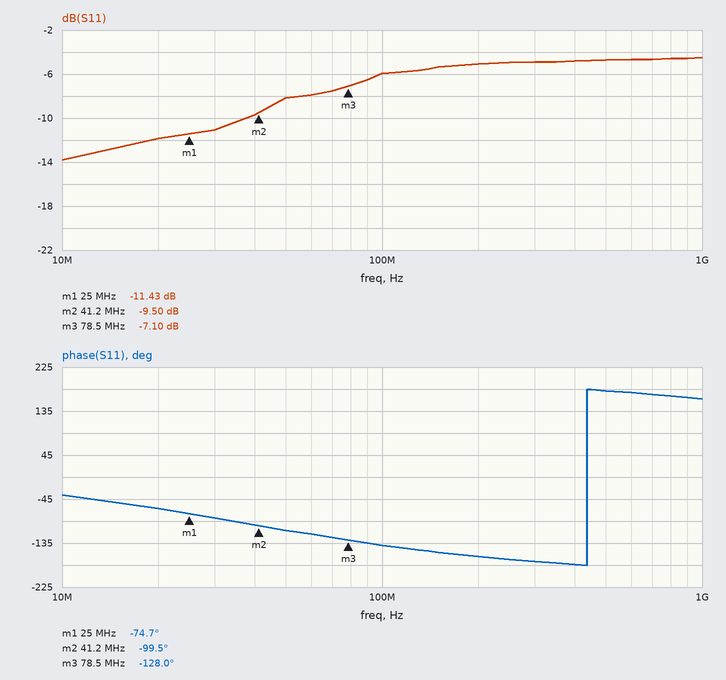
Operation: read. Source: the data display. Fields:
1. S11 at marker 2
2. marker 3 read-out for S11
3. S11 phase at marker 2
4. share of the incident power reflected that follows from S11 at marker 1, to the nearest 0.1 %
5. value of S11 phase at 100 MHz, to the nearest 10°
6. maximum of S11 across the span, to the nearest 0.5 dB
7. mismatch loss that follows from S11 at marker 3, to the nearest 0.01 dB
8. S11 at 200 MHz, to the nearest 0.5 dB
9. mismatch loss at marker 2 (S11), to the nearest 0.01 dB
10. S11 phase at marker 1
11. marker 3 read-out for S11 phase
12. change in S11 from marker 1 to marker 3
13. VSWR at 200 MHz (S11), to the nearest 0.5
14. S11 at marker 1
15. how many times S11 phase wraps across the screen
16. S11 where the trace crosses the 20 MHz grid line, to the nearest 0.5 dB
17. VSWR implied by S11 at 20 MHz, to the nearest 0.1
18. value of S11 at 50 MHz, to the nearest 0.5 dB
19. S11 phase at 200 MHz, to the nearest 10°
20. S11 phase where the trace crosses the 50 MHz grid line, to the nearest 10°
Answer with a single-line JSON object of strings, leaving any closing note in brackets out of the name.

{"S11 at marker 2": "-9.50 dB", "marker 3 read-out for S11": "-7.10 dB", "S11 phase at marker 2": "-99.5°", "share of the incident power reflected that follows from S11 at marker 1, to the nearest 0.1 %": "7.2 %", "value of S11 phase at 100 MHz, to the nearest 10°": "-140°", "maximum of S11 across the span, to the nearest 0.5 dB": "-4.5 dB", "mismatch loss that follows from S11 at marker 3, to the nearest 0.01 dB": "0.94 dB", "S11 at 200 MHz, to the nearest 0.5 dB": "-5.0 dB", "mismatch loss at marker 2 (S11), to the nearest 0.01 dB": "0.52 dB", "S11 phase at marker 1": "-74.7°", "marker 3 read-out for S11 phase": "-128.0°", "change in S11 from marker 1 to marker 3": "4.33 dB", "VSWR at 200 MHz (S11), to the nearest 0.5": "3.5", "S11 at marker 1": "-11.43 dB", "how many times S11 phase wraps across the screen": "1", "S11 where the trace crosses the 20 MHz grid line, to the nearest 0.5 dB": "-12.0 dB", "VSWR implied by S11 at 20 MHz, to the nearest 0.1": "1.7", "value of S11 at 50 MHz, to the nearest 0.5 dB": "-8.0 dB", "S11 phase at 200 MHz, to the nearest 10°": "-160°", "S11 phase where the trace crosses the 50 MHz grid line, to the nearest 10°": "-110°"}
